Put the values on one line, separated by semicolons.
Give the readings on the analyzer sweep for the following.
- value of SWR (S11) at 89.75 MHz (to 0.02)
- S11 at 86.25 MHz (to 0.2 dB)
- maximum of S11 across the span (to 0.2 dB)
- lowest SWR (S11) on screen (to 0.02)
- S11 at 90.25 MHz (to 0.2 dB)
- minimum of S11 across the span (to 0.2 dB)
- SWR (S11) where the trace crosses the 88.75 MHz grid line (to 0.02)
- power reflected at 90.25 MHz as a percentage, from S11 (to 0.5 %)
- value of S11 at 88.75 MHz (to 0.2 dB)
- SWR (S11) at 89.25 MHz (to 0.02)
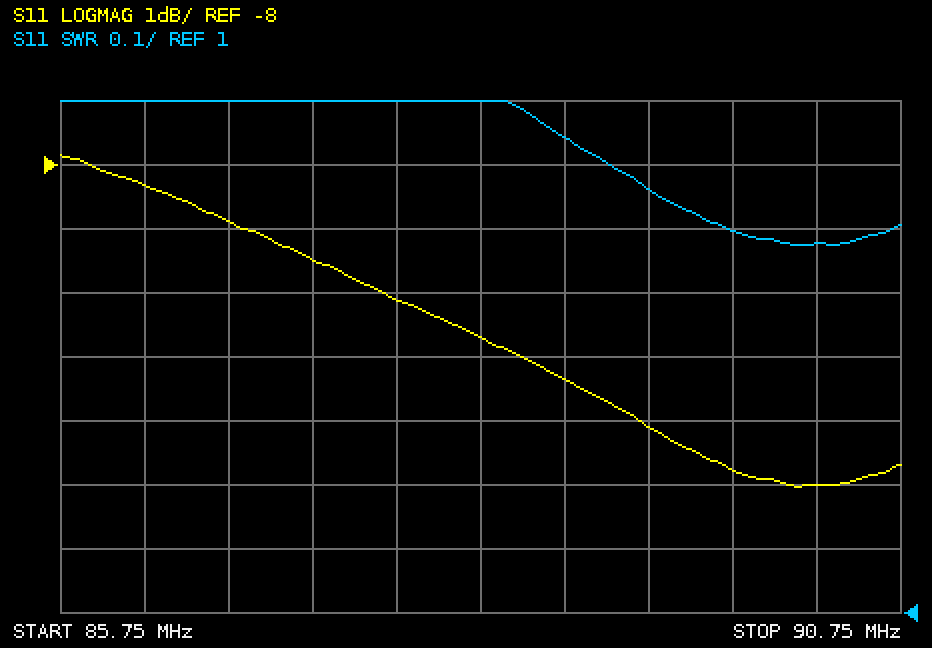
1.60; -8.4 dB; -7.8 dB; 1.58; -13.0 dB; -13.0 dB; 1.74; 5.0 %; -11.4 dB; 1.66
